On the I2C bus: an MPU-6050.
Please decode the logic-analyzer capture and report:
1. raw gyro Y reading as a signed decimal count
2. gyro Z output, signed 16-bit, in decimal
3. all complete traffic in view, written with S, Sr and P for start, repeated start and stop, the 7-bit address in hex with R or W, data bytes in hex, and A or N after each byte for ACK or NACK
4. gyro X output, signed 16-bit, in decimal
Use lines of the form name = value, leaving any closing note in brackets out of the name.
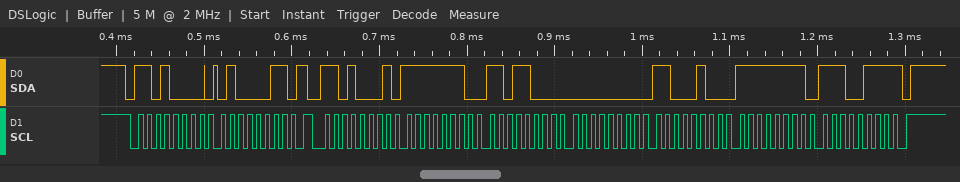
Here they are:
raw gyro Y reading as a signed decimal count = 196
gyro Z output, signed 16-bit, in decimal = -25
all complete traffic in view, written with S, Sr and P for start, repeated start and stop, the 7-bit address in hex with R or W, data bytes in hex, and A or N after each byte for ACK or NACK = S 68W A 43 A Sr 68R A FE A D8 A 00 A C4 A FF A E7 N P
gyro X output, signed 16-bit, in decimal = -296
